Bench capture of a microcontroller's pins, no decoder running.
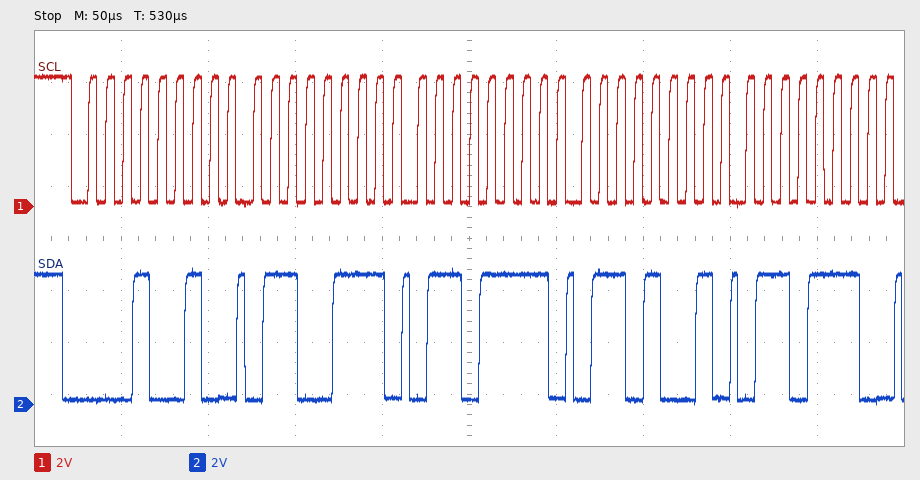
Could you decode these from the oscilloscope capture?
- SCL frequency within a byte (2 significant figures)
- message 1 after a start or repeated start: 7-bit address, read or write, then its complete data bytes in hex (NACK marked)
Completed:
100 kHz
0x09 write: 67 6F 69 6E
